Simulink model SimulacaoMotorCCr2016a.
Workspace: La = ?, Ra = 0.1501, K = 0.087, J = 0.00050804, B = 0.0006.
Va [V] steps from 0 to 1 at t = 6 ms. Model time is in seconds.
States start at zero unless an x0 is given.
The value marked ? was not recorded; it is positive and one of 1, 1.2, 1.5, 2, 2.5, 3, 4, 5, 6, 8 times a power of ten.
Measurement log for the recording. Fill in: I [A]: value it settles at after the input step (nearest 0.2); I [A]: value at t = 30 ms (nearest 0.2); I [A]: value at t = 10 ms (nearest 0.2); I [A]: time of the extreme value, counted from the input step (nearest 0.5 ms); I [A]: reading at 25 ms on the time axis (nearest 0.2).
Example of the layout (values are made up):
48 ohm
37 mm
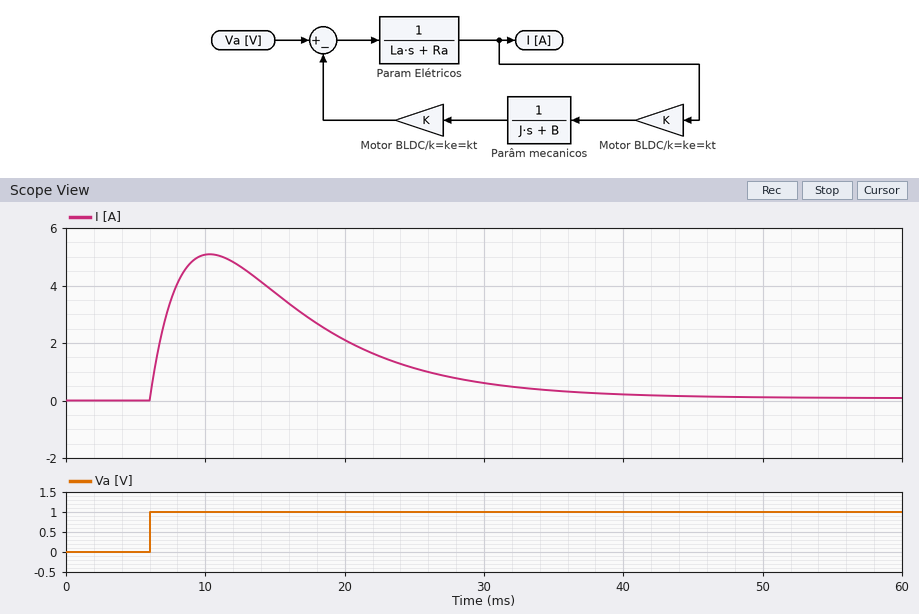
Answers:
0.0
0.6
5.0
4.5 ms
1.2
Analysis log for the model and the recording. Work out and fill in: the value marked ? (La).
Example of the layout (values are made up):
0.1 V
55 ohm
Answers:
0.0003
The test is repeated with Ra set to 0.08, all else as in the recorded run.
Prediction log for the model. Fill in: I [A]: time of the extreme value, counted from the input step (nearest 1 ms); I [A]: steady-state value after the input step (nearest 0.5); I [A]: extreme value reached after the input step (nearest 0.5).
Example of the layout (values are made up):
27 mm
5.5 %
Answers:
5 ms
0.0
7.5
